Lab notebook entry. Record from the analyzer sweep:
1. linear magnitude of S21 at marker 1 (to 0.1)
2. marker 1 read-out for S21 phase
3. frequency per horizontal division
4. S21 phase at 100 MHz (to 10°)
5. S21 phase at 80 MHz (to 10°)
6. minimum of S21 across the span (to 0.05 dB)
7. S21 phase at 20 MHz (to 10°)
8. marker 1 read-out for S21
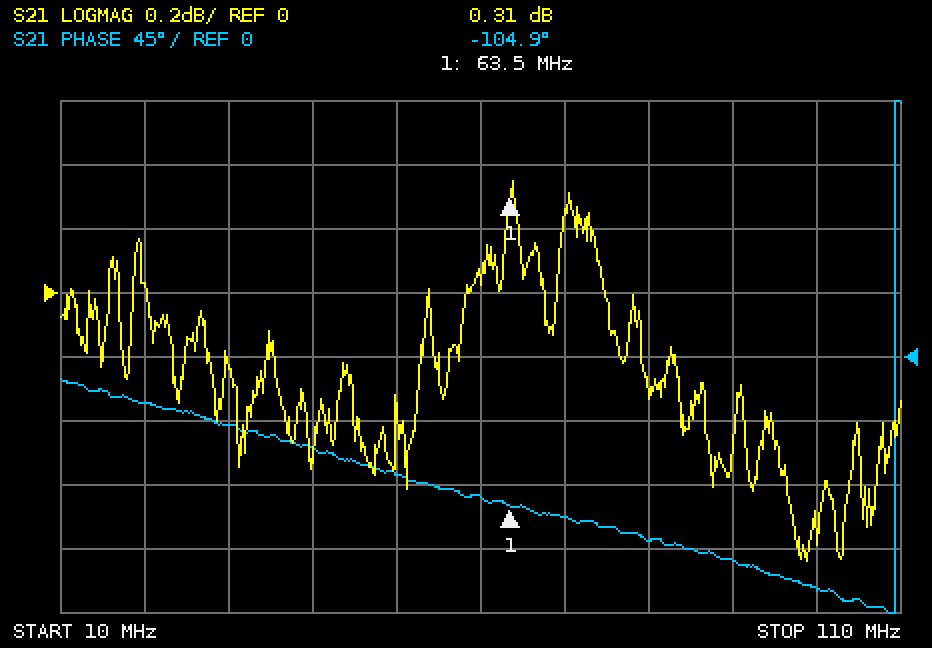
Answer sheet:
1.0
-104.9°
10 MHz
-160°
-130°
-0.85 dB
-30°
0.31 dB
